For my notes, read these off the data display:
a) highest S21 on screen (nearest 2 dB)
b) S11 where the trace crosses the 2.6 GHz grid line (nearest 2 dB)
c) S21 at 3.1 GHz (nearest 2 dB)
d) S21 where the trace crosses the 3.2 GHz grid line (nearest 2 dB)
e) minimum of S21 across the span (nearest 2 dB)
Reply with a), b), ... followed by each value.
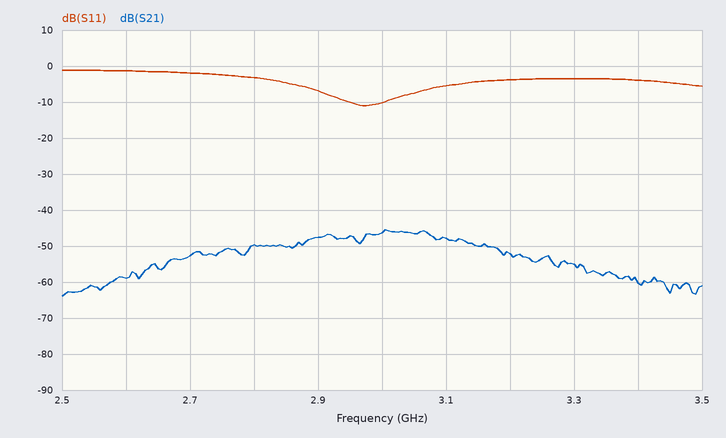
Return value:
a) -46 dB
b) -2 dB
c) -48 dB
d) -52 dB
e) -64 dB
